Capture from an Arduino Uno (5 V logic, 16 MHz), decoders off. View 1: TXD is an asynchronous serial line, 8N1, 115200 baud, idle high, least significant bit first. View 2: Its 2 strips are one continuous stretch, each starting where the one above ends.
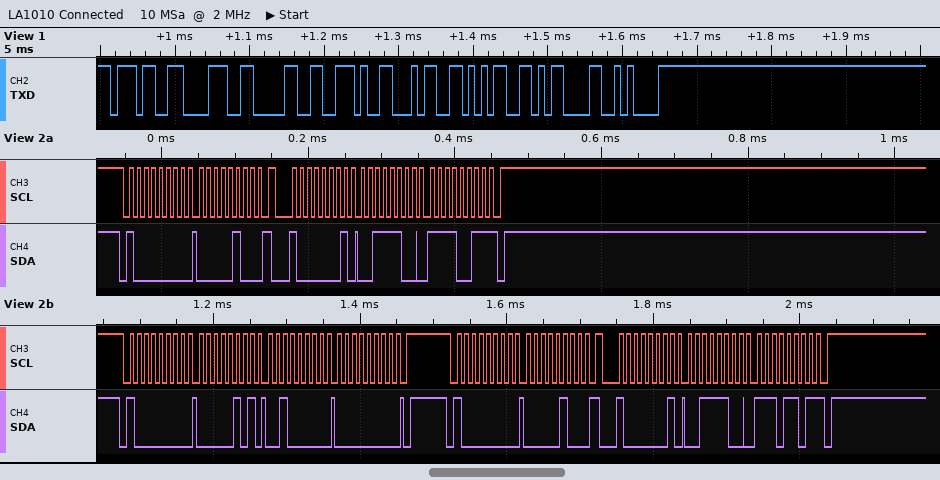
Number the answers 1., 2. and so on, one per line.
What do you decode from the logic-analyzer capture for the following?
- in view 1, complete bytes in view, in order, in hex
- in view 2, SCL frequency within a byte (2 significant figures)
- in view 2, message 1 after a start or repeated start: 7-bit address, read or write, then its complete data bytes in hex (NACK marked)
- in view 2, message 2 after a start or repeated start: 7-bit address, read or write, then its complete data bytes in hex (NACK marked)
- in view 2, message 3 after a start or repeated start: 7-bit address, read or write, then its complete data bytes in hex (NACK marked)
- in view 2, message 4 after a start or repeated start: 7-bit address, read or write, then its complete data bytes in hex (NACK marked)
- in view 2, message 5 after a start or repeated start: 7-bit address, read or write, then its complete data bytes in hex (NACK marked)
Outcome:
1. 37 38 30 2E 34 35 0D 0A
2. 100 kHz
3. 0x40 write: 04
4. 0x40 read: 3C F3 NACK
5. 0x40 write: 05 20 00
6. 0x40 write: 04
7. 0x40 read: 3C ED NACK
